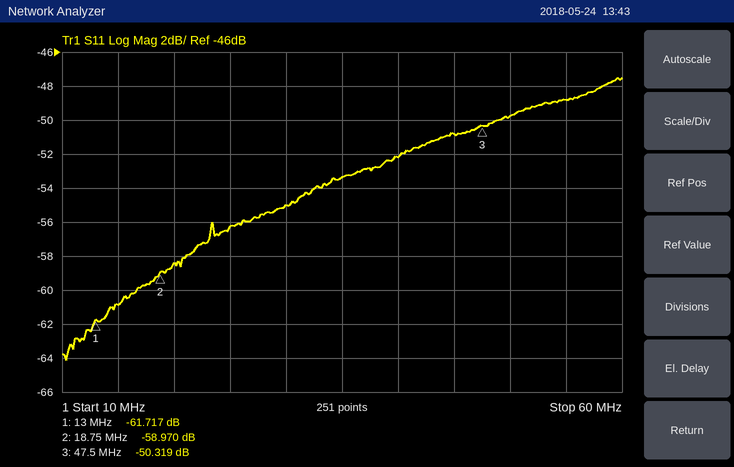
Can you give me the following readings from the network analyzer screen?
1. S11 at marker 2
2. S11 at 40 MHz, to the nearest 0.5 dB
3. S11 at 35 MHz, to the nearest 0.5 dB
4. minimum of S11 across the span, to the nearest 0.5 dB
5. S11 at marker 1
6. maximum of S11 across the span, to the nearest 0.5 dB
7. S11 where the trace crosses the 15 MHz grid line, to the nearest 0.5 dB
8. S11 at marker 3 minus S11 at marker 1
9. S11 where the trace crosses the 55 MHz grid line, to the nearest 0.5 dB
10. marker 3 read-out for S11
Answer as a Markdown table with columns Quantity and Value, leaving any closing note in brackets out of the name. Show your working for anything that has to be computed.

| Quantity | Value |
|---|---|
| S11 at marker 2 | -58.970 dB |
| S11 at 40 MHz, to the nearest 0.5 dB | -52.0 dB |
| S11 at 35 MHz, to the nearest 0.5 dB | -53.5 dB |
| minimum of S11 across the span, to the nearest 0.5 dB | -64.0 dB |
| S11 at marker 1 | -61.717 dB |
| maximum of S11 across the span, to the nearest 0.5 dB | -47.5 dB |
| S11 where the trace crosses the 15 MHz grid line, to the nearest 0.5 dB | -61.0 dB |
| S11 at marker 3 minus S11 at marker 1 | -50.319 − (-61.717) = 11.398 dB |
| S11 where the trace crosses the 55 MHz grid line, to the nearest 0.5 dB | -49.0 dB |
| marker 3 read-out for S11 | -50.319 dB |
